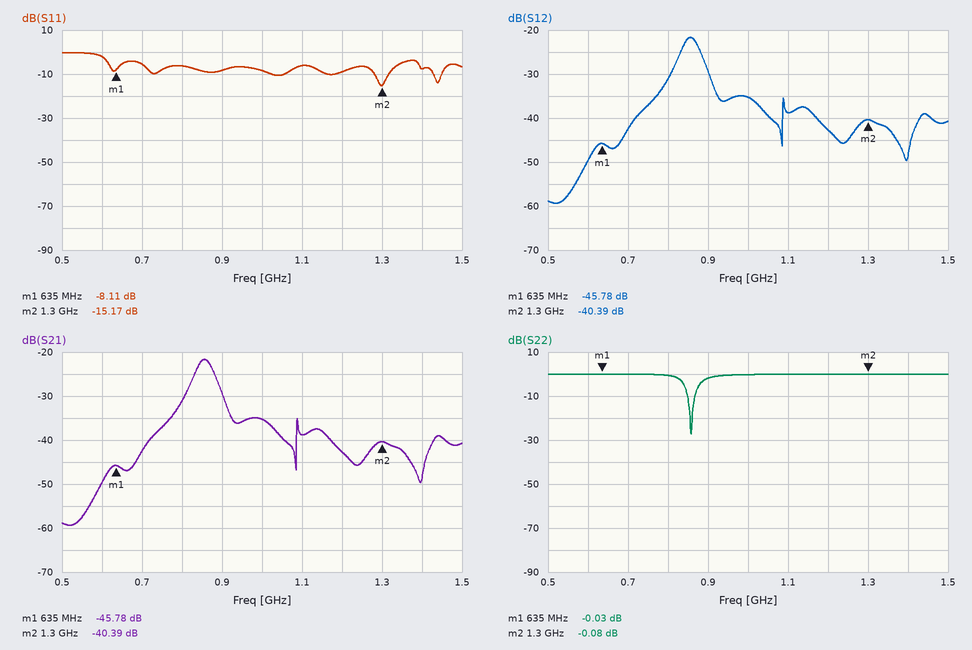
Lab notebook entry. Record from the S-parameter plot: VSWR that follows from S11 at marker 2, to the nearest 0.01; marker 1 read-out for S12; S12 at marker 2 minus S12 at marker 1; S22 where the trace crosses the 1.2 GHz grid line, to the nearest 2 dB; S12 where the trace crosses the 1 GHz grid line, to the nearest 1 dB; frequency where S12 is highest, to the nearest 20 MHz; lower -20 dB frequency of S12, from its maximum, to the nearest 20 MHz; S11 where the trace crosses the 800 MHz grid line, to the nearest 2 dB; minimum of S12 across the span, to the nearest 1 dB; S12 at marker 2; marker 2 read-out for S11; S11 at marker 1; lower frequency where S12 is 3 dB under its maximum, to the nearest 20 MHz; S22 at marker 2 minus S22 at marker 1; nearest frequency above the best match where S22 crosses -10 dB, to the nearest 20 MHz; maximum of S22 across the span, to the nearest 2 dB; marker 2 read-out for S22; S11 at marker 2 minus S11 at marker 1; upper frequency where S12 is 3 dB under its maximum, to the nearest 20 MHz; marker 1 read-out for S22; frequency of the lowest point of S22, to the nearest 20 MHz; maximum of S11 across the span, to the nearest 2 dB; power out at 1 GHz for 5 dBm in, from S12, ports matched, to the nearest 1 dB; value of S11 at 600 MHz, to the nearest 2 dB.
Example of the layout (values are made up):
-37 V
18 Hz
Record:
1.42
-45.78 dB
5.39 dB
0 dB
-35 dB
860 MHz
700 MHz
-6 dB
-59 dB
-40.39 dB
-15.17 dB
-8.11 dB
840 MHz
-0.05 dB
860 MHz
0 dB
-0.08 dB
-7.06 dB
880 MHz
-0.03 dB
860 MHz
0 dB
-30 dBm
-2 dB
